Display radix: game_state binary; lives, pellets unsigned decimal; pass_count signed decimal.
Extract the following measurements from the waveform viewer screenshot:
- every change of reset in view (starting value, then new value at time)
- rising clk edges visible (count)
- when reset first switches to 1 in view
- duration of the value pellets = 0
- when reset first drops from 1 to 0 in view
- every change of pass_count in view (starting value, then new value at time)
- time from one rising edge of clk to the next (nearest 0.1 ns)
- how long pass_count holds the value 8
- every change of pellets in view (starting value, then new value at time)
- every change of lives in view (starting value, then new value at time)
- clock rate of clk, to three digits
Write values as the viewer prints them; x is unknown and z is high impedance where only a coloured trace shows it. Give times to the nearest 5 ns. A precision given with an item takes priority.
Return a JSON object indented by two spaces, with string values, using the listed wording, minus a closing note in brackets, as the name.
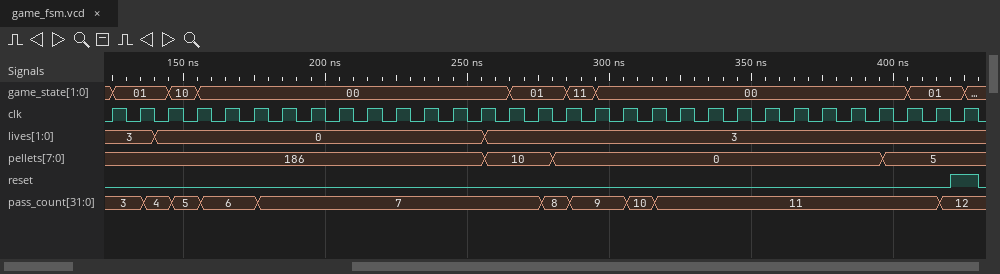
{
  "every change of reset in view": "0, 1 at 420 ns, 0 at 430 ns",
  "rising clk edges visible": "31",
  "when reset first switches to 1 in view": "420 ns",
  "duration of the value pellets = 0": "115 ns",
  "when reset first drops from 1 to 0 in view": "430 ns",
  "every change of pass_count in view": "3, 4 at 135 ns, 5 at 145 ns, 6 at 155 ns, 7 at 175 ns, 8 at 275 ns, 9 at 285 ns, 10 at 305 ns, 11 at 315 ns, 12 at 415 ns",
  "time from one rising edge of clk to the next": "10 ns",
  "how long pass_count holds the value 8": "10 ns",
  "every change of pellets in view": "186, 10 at 255 ns, 0 at 280 ns, 5 at 395 ns",
  "every change of lives in view": "3, 0 at 140 ns, 3 at 255 ns",
  "clock rate of clk, to three digits": "100 MHz"
}
